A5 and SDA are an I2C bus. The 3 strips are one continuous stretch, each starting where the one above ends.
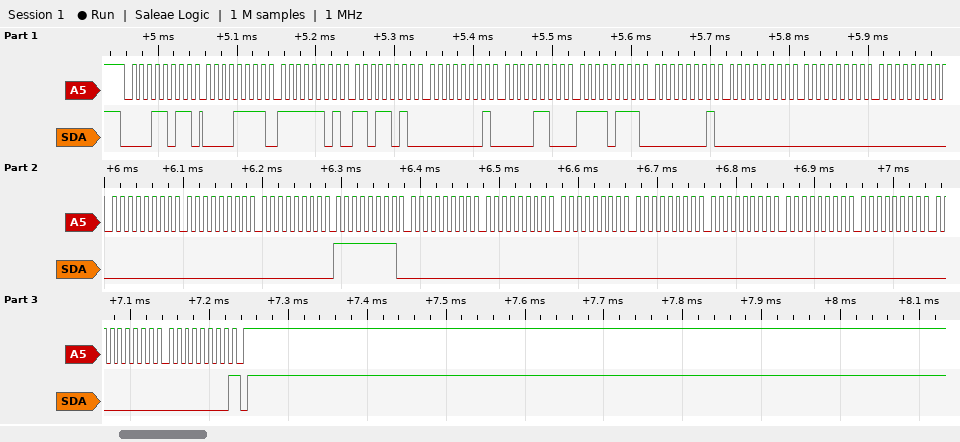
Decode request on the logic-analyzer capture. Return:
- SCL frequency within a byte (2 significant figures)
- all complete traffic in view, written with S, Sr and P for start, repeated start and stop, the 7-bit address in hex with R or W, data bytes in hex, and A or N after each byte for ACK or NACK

100 kHz
S 0DR A 0F A FD A DA A 01 A 0C A F7 A 01 A 00 A 00 A 00 A 00 A 00 A 00 A FF A 00 A 00 A 00 A 00 A 00 A 00 A 00 A 00 A 00 N P
